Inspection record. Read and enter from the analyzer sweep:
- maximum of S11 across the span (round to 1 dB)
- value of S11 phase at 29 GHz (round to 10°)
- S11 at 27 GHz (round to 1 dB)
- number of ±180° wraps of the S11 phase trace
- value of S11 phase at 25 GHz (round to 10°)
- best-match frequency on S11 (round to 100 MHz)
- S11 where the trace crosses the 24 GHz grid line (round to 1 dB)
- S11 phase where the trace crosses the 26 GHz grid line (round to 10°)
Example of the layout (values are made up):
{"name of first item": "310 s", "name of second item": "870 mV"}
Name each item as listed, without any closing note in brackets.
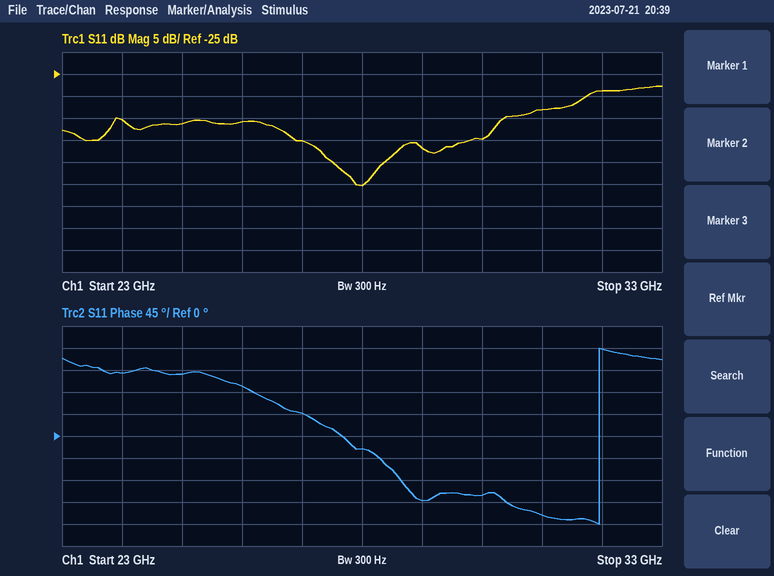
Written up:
{"maximum of S11 across the span": "-28 dB", "value of S11 phase at 29 GHz": "-130°", "S11 at 27 GHz": "-40 dB", "number of ±180° wraps of the S11 phase trace": "1", "value of S11 phase at 25 GHz": "130°", "best-match frequency on S11": "28.0 GHz", "S11 where the trace crosses the 24 GHz grid line": "-35 dB", "S11 phase where the trace crosses the 26 GHz grid line": "100°"}
